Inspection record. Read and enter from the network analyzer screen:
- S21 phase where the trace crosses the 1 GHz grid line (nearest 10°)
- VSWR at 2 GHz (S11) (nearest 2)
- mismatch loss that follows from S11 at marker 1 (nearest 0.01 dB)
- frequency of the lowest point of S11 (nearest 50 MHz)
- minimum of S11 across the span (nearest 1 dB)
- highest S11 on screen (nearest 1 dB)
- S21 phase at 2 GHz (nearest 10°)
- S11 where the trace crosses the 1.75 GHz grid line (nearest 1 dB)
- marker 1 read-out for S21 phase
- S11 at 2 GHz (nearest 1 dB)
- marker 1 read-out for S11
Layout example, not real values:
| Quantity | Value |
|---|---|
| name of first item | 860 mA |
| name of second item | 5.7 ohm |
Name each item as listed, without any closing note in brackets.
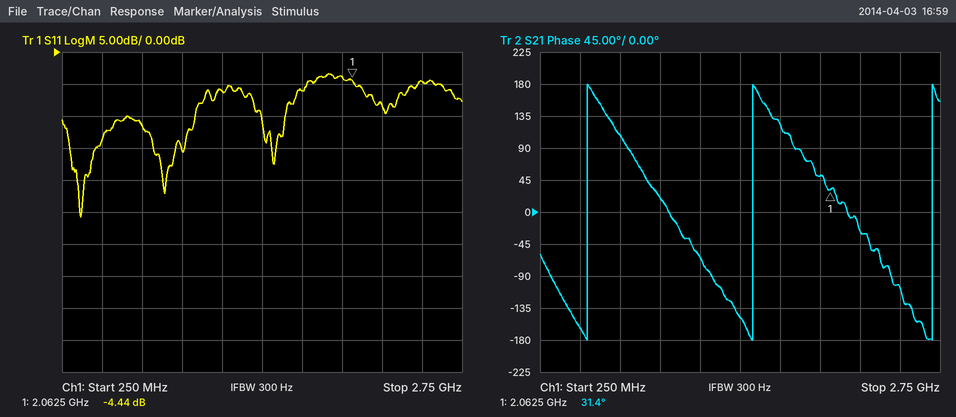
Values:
| Quantity | Value |
|---|---|
| S21 phase where the trace crosses the 1 GHz grid line | 20° |
| VSWR at 2 GHz (S11) | 4 |
| mismatch loss that follows from S11 at marker 1 | 1.94 dB |
| frequency of the lowest point of S11 | 350 MHz |
| minimum of S11 across the span | -26 dB |
| highest S11 on screen | -3 dB |
| S21 phase at 2 GHz | 50° |
| S11 where the trace crosses the 1.75 GHz grid line | -6 dB |
| marker 1 read-out for S21 phase | 31.4° |
| S11 at 2 GHz | -4 dB |
| marker 1 read-out for S11 | -4.44 dB |
